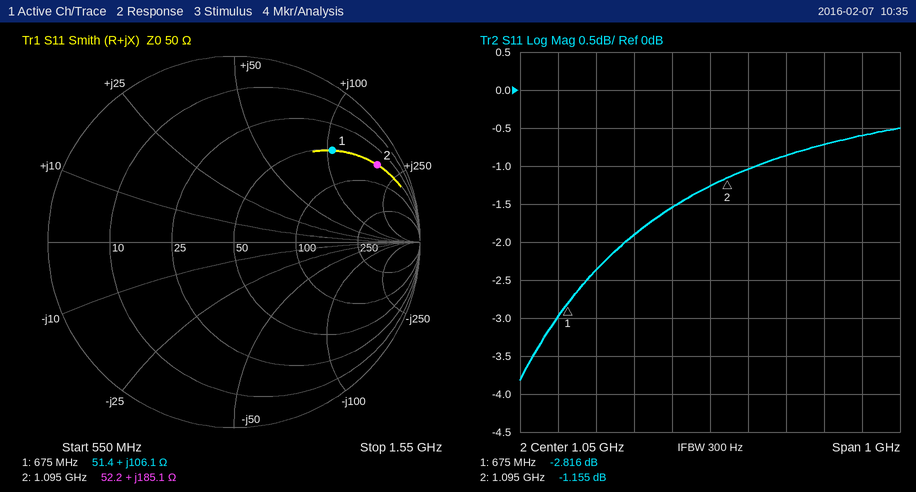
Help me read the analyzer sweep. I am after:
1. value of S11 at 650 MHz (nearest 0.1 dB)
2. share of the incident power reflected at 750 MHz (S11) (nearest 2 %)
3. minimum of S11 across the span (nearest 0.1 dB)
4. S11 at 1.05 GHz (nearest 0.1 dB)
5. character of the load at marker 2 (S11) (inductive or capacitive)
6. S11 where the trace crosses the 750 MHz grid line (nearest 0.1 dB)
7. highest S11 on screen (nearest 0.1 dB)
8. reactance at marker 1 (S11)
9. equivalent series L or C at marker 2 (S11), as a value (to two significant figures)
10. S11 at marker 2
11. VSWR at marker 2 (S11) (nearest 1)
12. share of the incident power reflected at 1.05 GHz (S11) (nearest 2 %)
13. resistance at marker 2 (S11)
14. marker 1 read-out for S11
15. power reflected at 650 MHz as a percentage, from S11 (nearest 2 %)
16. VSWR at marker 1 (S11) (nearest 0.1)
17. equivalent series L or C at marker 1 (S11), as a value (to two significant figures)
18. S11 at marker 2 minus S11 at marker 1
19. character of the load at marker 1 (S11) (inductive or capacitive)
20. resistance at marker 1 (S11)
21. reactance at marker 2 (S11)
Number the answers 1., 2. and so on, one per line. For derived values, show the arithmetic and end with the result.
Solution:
1. -3.0 dB
2. 10^(-2.4/10) ≈ 58 %
3. -3.8 dB
4. -1.3 dB
5. inductive
6. -2.4 dB
7. -0.5 dB
8. +106.1 Ω
9. L = 185.1 Ω/(2π × 1.095 GHz) ≈ 27 nH
10. -1.155 dB
11. 15
12. 10^(-1.3/10) ≈ 74 %
13. 52.2 Ω
14. -2.816 dB
15. 10^(-3/10) ≈ 50 %
16. 6.2
17. L = 106.1 Ω/(2π × 675 MHz) ≈ 25 nH
18. -1.155 − (-2.816) = 1.661 dB
19. inductive
20. 51.4 Ω
21. +185.1 Ω
